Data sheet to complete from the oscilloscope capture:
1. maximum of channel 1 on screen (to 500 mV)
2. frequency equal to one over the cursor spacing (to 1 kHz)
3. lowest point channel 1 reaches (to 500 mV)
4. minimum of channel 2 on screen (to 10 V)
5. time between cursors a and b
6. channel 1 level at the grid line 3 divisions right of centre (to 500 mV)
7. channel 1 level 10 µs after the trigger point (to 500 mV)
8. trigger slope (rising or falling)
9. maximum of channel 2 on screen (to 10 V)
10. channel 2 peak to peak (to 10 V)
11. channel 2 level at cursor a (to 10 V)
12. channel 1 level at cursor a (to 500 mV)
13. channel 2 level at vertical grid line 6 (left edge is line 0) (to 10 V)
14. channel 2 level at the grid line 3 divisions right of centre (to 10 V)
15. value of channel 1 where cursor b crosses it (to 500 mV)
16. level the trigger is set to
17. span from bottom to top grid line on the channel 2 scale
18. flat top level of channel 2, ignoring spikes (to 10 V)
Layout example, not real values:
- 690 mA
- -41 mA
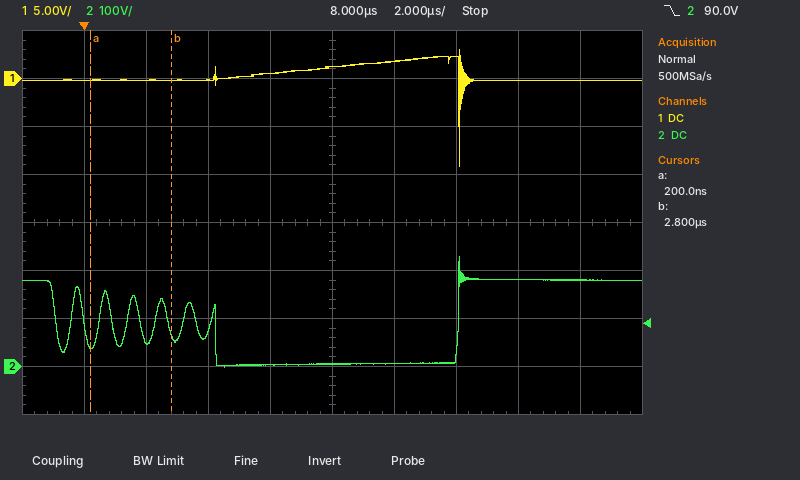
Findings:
- 3.0 V
- 385 kHz
- -9.0 V
- 0 V
- 2.6 µs
- 0.0 V
- 2.0 V
- falling
- 230 V
- 230 V
- 50 V
- 0.0 V
- 10 V
- 180 V
- 0.0 V
- 90.0 V
- 800 V
- 180 V
